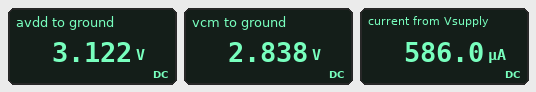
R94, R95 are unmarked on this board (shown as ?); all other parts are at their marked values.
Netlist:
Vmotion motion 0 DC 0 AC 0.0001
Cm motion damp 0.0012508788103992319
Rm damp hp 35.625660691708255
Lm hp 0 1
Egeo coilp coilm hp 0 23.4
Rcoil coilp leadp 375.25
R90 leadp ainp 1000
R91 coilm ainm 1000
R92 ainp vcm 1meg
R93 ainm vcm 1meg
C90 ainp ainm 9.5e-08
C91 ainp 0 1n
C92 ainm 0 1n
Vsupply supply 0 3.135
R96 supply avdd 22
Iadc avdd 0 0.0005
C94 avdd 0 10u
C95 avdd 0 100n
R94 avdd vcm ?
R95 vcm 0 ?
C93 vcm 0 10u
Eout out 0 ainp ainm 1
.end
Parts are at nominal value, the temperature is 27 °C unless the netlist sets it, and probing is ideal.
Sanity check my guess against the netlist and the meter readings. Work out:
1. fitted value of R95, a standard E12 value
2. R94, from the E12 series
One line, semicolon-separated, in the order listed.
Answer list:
33 kΩ; 3.3 kΩ
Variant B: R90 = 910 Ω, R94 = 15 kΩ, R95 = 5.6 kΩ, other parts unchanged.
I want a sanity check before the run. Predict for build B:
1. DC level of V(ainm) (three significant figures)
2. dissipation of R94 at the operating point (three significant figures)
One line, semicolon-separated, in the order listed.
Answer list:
848 mV; 344 µW
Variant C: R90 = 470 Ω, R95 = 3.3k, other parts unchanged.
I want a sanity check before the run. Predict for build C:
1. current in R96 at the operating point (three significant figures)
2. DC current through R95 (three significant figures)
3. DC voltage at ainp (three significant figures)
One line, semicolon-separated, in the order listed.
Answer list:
972 µA; 472 µA; 1.56 V
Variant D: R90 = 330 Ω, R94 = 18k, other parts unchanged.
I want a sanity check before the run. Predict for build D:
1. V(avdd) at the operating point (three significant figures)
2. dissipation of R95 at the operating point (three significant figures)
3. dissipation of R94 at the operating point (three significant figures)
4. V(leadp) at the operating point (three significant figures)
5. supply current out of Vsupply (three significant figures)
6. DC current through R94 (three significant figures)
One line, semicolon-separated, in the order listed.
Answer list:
3.12 V; 124 µW; 67.5 µW; 2.02 V; 561 µA; 61.2 µA
